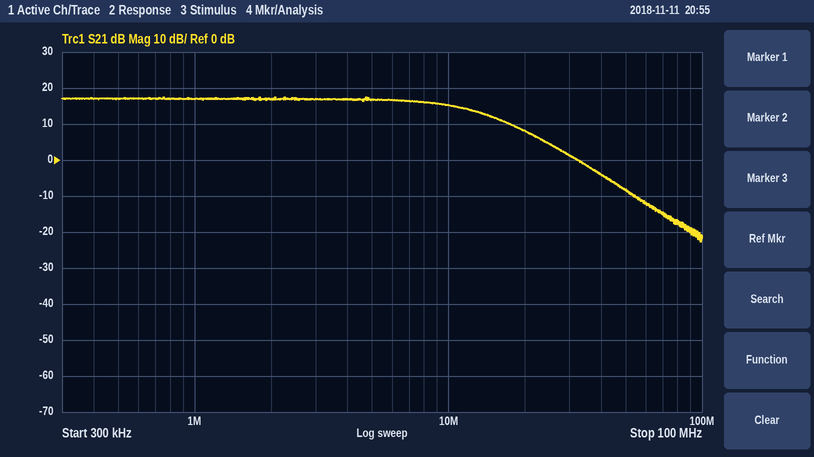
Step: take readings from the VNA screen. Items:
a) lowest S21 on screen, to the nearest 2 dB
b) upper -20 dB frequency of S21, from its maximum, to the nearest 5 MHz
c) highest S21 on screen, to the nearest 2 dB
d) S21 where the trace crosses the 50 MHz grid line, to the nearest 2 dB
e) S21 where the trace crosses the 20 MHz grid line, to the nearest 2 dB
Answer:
-22 dB
35 MHz
18 dB
-8 dB
8 dB
